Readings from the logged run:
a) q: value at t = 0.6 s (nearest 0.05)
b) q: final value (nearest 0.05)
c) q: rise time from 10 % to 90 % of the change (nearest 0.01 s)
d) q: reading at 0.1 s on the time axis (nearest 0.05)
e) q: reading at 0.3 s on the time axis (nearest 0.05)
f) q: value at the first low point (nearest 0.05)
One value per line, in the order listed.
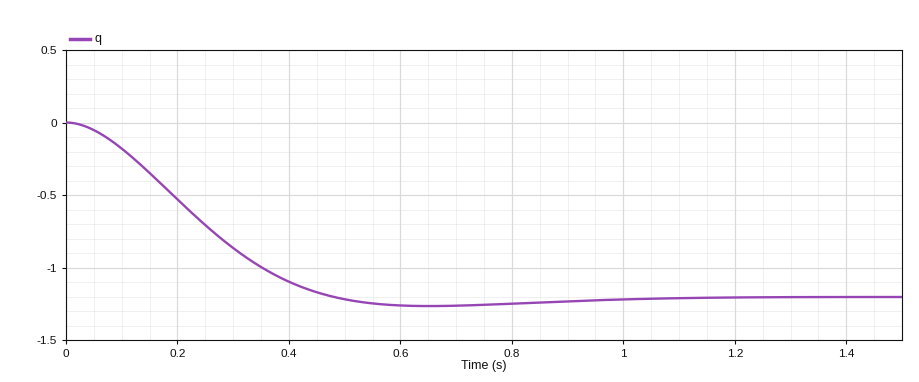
-1.25
-1.20
0.31 s
-0.20
-0.85
-1.25
